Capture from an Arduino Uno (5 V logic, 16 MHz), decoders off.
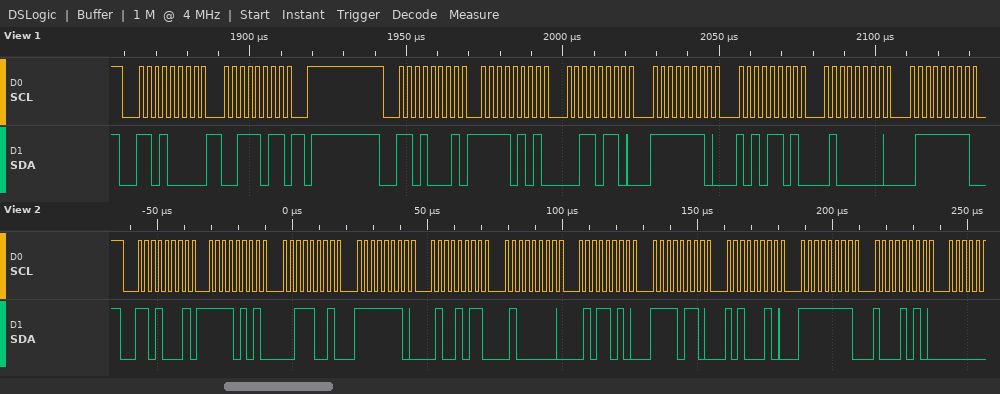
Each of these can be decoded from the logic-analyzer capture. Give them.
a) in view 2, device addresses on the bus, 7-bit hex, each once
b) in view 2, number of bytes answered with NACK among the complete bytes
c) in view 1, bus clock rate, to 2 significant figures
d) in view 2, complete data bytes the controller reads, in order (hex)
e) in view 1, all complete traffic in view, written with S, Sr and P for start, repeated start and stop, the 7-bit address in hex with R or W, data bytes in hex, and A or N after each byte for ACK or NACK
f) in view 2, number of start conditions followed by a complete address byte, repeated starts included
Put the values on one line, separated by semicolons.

0x68; 0; 400 kHz; F5 39 FE 4B 40 5A F6 A2 FF 8A; S 68W A 3B A P S 68R A F5 A 36 A FE A AD A 40 A 7F A; 1
